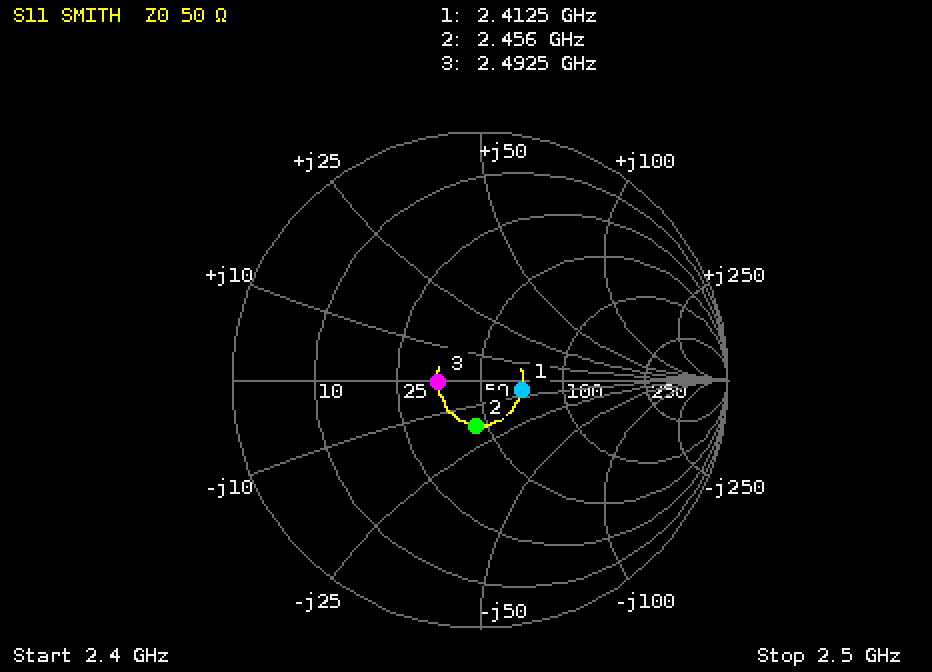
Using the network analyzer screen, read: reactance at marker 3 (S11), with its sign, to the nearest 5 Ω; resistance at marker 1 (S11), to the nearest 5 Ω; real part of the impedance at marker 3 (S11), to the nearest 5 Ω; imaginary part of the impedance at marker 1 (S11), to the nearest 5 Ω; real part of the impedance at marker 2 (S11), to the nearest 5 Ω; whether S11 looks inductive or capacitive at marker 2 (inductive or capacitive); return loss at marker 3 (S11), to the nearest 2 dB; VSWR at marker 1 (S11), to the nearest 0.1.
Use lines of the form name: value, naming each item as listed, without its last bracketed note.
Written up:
reactance at marker 3 (S11), with its sign, to the nearest 5 Ω: 0 Ω
resistance at marker 1 (S11), to the nearest 5 Ω: 70 Ω
real part of the impedance at marker 3 (S11), to the nearest 5 Ω: 35 Ω
imaginary part of the impedance at marker 1 (S11), to the nearest 5 Ω: -5 Ω
real part of the impedance at marker 2 (S11), to the nearest 5 Ω: 45 Ω
whether S11 looks inductive or capacitive at marker 2: capacitive
return loss at marker 3 (S11), to the nearest 2 dB: 16 dB
VSWR at marker 1 (S11), to the nearest 0.1: 1.4
